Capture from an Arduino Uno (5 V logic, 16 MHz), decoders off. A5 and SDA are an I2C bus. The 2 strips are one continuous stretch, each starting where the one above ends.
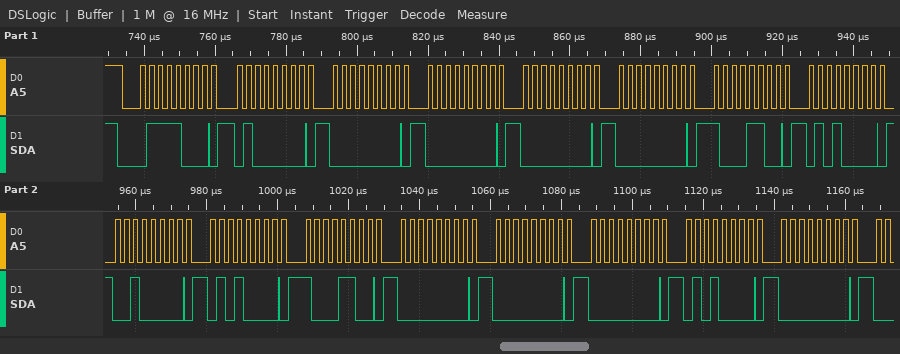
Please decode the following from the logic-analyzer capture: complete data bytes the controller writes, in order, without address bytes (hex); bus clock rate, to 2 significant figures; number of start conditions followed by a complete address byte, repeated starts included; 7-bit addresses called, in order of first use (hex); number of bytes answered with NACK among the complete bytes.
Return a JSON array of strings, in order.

["40 00 00 00 00 8C 50 20 50 8C 00 00 00 50 00", "400 kHz", "1", "0x3C", "0"]
